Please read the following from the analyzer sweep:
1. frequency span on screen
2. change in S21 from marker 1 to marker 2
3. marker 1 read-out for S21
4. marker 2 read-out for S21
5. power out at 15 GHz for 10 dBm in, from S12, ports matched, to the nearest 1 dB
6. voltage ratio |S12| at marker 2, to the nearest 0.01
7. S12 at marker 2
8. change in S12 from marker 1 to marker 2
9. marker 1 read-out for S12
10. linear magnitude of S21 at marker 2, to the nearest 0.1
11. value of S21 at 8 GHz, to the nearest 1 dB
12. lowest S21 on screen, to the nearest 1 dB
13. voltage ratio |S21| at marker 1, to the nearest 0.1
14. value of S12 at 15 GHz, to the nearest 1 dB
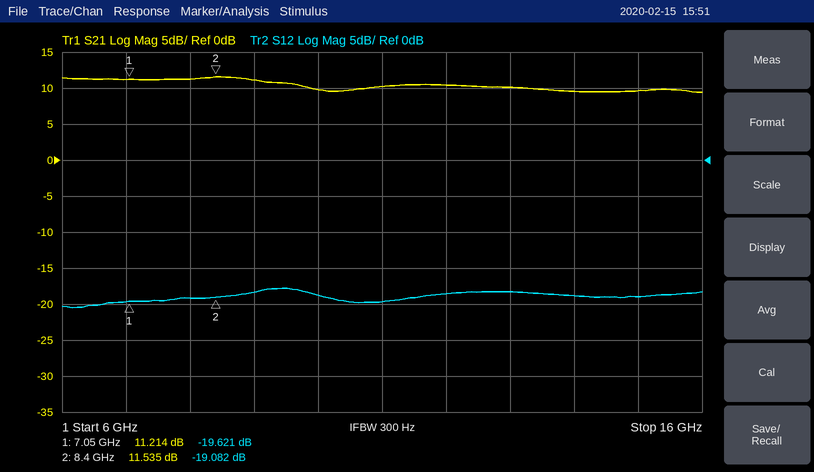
10 GHz
0.321 dB
11.214 dB
11.535 dB
-9 dBm
0.11
-19.082 dB
0.539 dB
-19.621 dB
3.8
11 dB
9 dB
3.6
-19 dB
